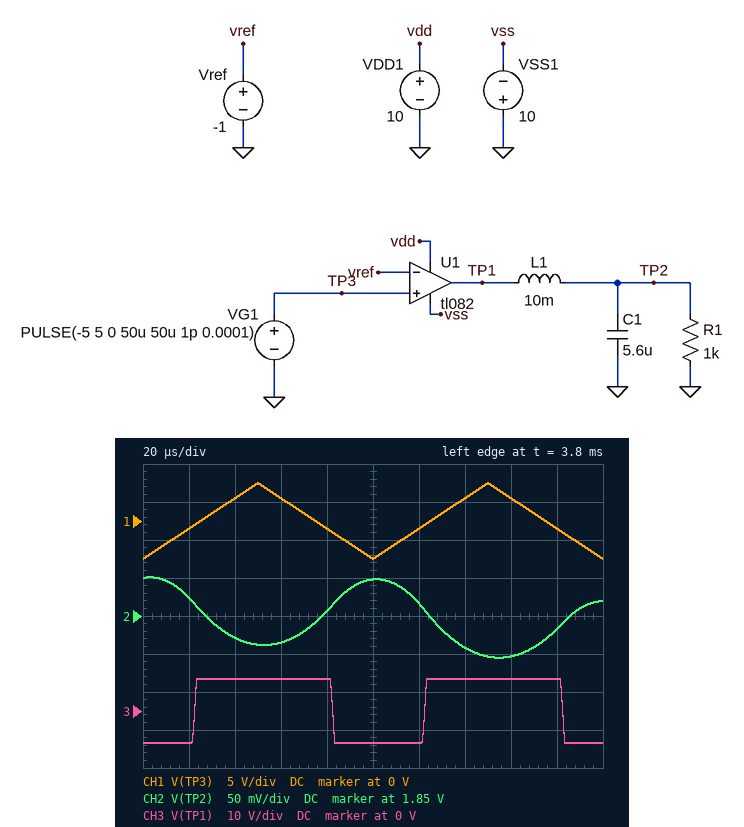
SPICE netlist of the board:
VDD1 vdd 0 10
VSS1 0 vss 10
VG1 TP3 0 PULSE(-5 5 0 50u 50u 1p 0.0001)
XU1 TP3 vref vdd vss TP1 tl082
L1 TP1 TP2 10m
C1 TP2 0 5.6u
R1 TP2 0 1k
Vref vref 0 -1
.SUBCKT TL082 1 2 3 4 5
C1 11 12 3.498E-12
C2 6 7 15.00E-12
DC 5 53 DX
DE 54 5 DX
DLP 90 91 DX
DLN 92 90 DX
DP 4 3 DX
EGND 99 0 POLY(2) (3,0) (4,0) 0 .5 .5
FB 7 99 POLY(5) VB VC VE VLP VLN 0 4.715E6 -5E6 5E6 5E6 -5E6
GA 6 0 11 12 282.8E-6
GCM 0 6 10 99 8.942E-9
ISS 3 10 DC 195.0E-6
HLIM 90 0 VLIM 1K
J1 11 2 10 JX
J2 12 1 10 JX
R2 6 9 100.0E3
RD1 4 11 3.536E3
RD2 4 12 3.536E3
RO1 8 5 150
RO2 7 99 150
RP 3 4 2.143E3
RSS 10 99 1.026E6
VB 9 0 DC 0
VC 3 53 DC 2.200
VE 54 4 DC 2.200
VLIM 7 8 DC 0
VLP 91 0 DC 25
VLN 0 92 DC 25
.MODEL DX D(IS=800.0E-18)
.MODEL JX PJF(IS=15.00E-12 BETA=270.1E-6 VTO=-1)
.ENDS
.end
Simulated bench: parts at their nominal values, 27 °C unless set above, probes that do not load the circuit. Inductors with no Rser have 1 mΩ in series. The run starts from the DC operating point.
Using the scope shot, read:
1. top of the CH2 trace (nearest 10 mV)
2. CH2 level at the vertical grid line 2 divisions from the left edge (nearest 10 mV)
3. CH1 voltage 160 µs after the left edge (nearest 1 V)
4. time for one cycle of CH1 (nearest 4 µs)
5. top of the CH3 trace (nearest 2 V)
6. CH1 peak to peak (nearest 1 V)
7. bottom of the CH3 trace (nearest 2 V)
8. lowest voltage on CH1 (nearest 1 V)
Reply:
1.90 V
1.82 V
3 V
100 µs
8 V
10 V
-8 V
-5 V
